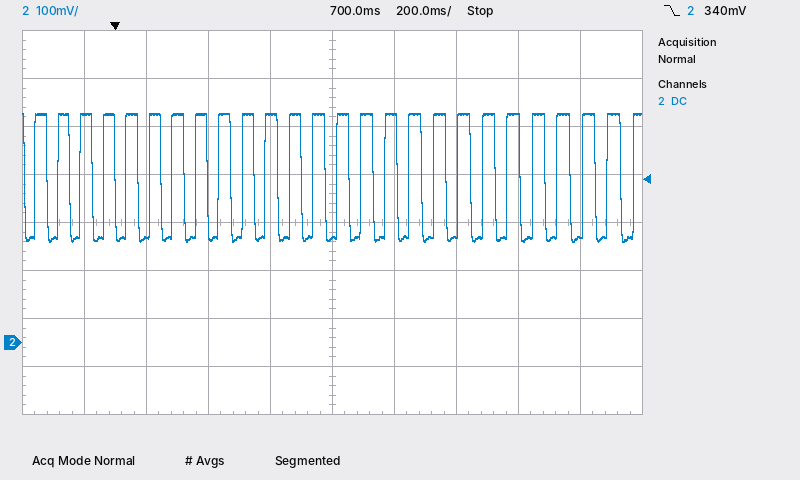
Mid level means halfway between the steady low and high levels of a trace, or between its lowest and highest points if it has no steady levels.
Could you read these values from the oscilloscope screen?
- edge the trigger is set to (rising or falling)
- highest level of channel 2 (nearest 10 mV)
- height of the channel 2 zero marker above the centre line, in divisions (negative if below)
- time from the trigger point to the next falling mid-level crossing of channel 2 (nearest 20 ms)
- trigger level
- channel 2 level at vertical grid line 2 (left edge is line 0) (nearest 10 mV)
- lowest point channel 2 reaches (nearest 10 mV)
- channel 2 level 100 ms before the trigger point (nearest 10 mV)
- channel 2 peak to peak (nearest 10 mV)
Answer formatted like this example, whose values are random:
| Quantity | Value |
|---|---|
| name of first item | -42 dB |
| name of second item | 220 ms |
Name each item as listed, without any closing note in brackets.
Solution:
| Quantity | Value |
|---|---|
| edge the trigger is set to | falling |
| highest level of channel 2 | 480 mV |
| height of the channel 2 zero marker above the centre line, in divisions | -2.5 div |
| time from the trigger point to the next falling mid-level crossing of channel 2 | 80 ms |
| trigger level | 340 mV |
| channel 2 level at vertical grid line 2 (left edge is line 0) | 220 mV |
| lowest point channel 2 reaches | 210 mV |
| channel 2 level 100 ms before the trigger point | 480 mV |
| channel 2 peak to peak | 270 mV |
